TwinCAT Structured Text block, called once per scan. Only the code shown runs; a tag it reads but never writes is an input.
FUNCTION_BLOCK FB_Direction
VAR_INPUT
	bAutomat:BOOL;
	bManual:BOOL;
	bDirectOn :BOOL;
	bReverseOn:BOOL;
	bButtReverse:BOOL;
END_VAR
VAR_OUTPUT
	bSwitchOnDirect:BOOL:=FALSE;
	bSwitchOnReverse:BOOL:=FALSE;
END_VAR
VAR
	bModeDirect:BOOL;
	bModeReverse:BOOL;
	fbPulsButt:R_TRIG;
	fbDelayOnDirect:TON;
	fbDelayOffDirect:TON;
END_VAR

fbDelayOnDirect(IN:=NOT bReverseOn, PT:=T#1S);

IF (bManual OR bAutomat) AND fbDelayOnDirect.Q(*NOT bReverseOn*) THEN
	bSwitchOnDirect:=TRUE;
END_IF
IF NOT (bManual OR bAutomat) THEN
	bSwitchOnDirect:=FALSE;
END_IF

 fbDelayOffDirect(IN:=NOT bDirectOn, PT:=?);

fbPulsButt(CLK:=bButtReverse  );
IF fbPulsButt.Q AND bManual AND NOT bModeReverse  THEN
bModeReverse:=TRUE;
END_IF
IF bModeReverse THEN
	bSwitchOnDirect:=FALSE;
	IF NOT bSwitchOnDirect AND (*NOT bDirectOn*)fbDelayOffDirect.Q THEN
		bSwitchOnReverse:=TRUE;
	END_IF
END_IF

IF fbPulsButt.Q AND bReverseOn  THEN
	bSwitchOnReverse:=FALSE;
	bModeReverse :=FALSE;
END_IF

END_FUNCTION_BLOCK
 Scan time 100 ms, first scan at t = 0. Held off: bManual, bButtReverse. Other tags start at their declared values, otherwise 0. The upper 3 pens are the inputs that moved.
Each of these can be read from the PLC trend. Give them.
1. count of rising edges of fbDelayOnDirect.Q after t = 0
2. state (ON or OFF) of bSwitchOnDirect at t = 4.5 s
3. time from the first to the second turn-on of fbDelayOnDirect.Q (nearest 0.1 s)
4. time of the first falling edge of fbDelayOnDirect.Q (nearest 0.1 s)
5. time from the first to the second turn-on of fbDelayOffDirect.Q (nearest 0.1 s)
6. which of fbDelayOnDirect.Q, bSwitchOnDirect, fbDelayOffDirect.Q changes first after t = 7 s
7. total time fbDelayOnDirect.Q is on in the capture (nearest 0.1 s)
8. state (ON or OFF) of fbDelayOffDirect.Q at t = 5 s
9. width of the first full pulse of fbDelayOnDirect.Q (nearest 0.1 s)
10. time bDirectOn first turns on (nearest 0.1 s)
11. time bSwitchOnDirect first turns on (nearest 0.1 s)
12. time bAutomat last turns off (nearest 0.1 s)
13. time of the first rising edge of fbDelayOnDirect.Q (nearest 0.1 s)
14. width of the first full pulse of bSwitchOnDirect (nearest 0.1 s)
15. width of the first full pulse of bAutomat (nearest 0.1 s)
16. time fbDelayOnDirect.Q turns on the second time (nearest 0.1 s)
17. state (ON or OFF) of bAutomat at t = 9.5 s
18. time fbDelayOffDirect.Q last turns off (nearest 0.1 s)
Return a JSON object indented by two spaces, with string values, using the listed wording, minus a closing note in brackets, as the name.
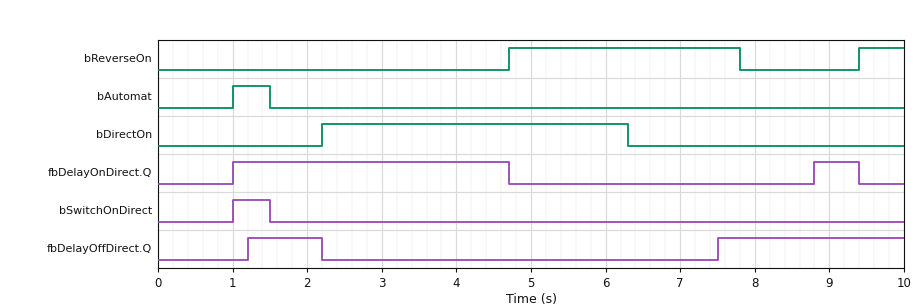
{
  "count of rising edges of fbDelayOnDirect.Q after t = 0": "2",
  "state (ON or OFF) of bSwitchOnDirect at t = 4.5 s": "OFF",
  "time from the first to the second turn-on of fbDelayOnDirect.Q": "7.8 s",
  "time of the first falling edge of fbDelayOnDirect.Q": "4.7 s",
  "time from the first to the second turn-on of fbDelayOffDirect.Q": "6.3 s",
  "which of fbDelayOnDirect.Q, bSwitchOnDirect, fbDelayOffDirect.Q changes first after t = 7 s": "fbDelayOffDirect.Q",
  "total time fbDelayOnDirect.Q is on in the capture": "4.3 s",
  "state (ON or OFF) of fbDelayOffDirect.Q at t = 5 s": "OFF",
  "width of the first full pulse of fbDelayOnDirect.Q": "3.7 s",
  "time bDirectOn first turns on": "2.2 s",
  "time bSwitchOnDirect first turns on": "1.0 s",
  "time bAutomat last turns off": "1.5 s",
  "time of the first rising edge of fbDelayOnDirect.Q": "1.0 s",
  "width of the first full pulse of bSwitchOnDirect": "0.5 s",
  "width of the first full pulse of bAutomat": "0.5 s",
  "time fbDelayOnDirect.Q turns on the second time": "8.8 s",
  "state (ON or OFF) of bAutomat at t = 9.5 s": "OFF",
  "time fbDelayOffDirect.Q last turns off": "2.2 s"
}
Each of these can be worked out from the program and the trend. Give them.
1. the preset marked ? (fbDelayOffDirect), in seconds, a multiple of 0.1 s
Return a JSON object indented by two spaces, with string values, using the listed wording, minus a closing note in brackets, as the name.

{
  "the preset marked ? (fbDelayOffDirect), in seconds, a multiple of 0.1 s": "1.2 s"
}
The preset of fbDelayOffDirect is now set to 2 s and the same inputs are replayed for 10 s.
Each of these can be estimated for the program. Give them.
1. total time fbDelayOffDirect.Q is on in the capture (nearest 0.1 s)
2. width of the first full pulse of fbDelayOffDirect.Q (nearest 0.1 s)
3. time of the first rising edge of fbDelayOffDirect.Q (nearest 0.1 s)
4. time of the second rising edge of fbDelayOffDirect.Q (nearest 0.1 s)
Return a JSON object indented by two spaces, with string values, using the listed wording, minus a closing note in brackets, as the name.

{
  "total time fbDelayOffDirect.Q is on in the capture": "1.9 s",
  "width of the first full pulse of fbDelayOffDirect.Q": "0.2 s",
  "time of the first rising edge of fbDelayOffDirect.Q": "2.0 s",
  "time of the second rising edge of fbDelayOffDirect.Q": "8.3 s"
}
